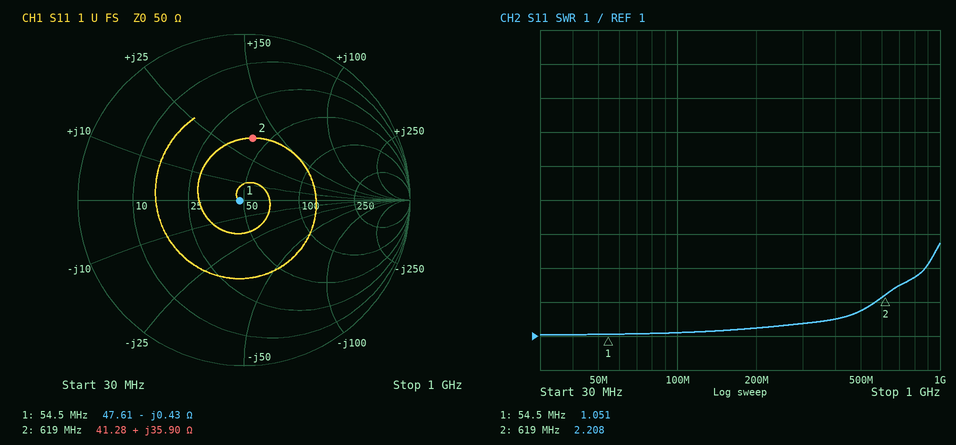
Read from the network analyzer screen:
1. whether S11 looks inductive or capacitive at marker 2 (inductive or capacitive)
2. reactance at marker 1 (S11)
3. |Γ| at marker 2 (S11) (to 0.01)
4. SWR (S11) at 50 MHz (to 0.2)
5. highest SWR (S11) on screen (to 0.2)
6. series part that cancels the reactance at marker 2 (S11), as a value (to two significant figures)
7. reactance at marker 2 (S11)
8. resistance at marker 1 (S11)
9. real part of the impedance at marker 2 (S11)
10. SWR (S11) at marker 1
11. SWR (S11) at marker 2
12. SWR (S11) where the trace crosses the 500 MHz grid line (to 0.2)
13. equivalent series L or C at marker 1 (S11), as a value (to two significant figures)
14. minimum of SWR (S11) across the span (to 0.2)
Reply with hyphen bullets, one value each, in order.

- inductive
- -0.43 Ω
- 0.38
- 1.0
- 3.8
- 7.2 pF
- +35.90 Ω
- 47.61 Ω
- 41.28 Ω
- 1.051
- 2.208
- 1.8
- 6.8 nF
- 1.0
